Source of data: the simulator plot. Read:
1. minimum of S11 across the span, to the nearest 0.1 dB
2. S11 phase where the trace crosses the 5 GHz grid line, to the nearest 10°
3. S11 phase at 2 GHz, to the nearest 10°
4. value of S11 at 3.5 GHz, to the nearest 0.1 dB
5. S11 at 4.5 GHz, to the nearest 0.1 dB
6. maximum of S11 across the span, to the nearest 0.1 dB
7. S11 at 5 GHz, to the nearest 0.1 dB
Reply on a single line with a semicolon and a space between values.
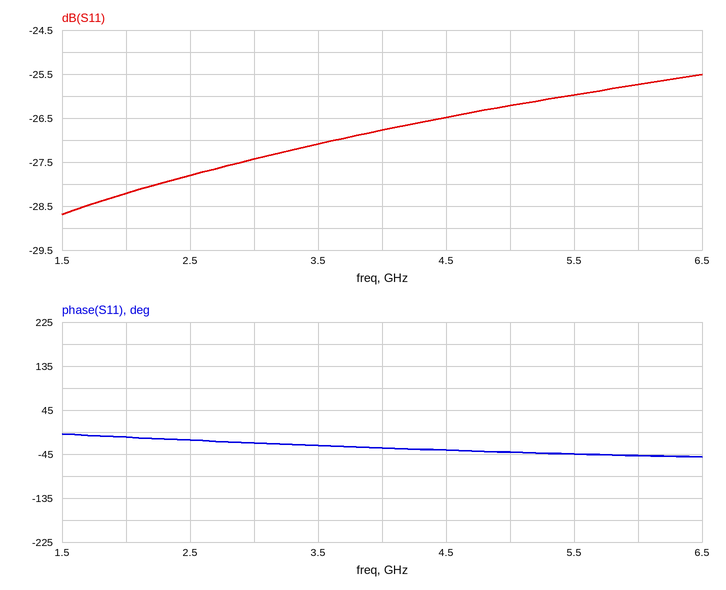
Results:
-28.7 dB; -40°; -10°; -27.1 dB; -26.5 dB; -25.5 dB; -26.2 dB
